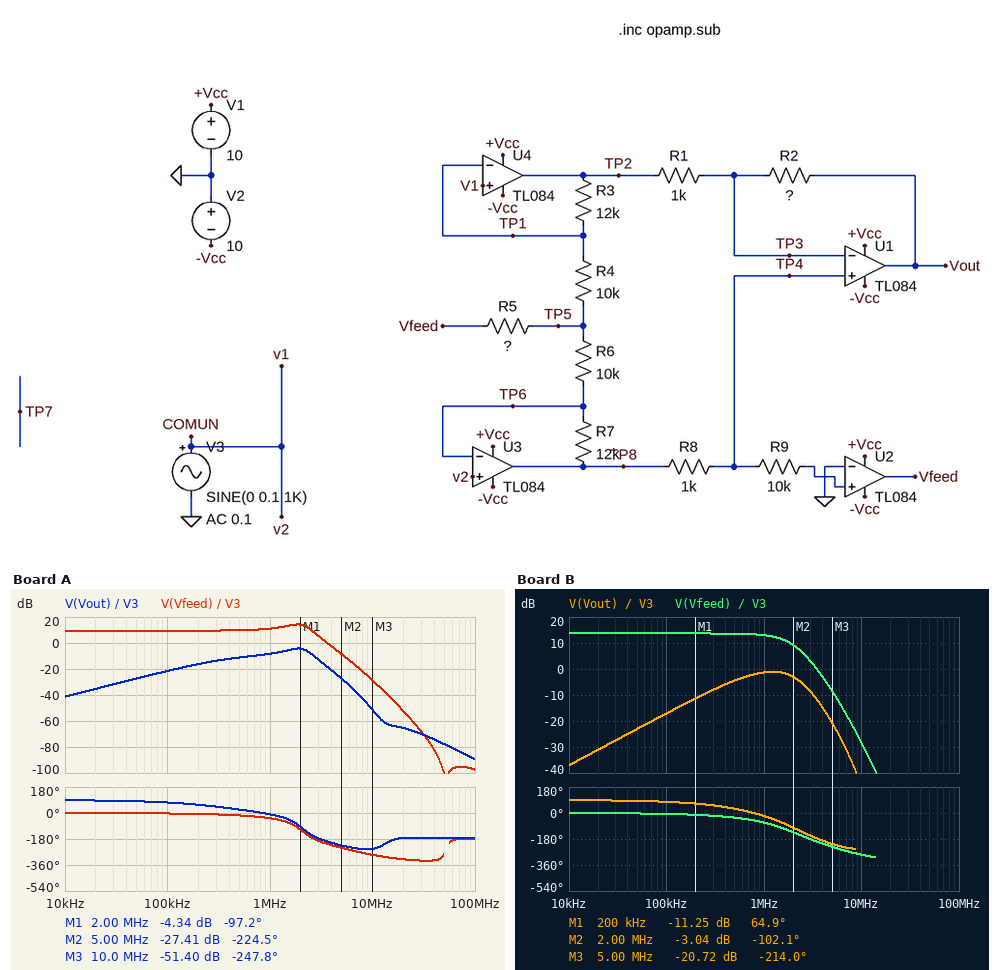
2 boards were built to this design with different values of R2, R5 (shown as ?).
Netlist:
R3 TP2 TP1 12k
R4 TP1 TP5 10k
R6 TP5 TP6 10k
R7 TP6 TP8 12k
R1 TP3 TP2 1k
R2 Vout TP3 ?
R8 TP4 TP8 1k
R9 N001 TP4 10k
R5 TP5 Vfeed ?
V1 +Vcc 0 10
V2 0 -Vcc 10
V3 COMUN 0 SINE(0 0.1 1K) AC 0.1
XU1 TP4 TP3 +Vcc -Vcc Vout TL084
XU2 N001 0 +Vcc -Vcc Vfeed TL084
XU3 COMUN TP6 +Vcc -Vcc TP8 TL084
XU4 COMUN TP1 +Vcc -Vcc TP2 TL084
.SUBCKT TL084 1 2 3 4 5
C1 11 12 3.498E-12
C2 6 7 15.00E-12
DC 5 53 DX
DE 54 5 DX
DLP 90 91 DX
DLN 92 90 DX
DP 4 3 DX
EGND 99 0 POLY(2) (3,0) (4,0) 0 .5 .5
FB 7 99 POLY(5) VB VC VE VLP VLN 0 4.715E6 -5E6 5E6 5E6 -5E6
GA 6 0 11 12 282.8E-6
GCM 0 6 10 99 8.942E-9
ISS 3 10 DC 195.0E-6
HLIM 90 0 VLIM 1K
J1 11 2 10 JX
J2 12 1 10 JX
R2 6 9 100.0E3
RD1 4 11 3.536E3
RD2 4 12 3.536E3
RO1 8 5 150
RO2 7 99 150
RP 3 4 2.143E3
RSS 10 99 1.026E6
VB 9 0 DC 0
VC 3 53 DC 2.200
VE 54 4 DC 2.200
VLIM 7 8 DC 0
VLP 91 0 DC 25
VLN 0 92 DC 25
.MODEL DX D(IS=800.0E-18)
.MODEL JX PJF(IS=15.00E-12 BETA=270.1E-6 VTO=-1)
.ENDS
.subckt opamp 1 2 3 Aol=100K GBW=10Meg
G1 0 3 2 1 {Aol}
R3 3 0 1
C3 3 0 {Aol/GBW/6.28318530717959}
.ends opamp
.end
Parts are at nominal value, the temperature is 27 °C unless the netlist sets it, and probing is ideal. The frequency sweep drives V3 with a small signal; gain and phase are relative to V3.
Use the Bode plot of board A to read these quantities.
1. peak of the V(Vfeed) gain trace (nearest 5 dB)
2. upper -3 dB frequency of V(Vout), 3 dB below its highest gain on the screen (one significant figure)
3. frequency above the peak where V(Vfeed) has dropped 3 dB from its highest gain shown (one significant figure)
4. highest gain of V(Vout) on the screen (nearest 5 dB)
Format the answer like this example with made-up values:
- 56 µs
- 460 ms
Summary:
- 15 dB
- 2 MHz
- 2 MHz
- -5 dB
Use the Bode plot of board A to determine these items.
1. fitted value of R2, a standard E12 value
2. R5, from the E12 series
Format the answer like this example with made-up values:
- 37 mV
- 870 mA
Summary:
- 8.2 kΩ
- 6.8 kΩ
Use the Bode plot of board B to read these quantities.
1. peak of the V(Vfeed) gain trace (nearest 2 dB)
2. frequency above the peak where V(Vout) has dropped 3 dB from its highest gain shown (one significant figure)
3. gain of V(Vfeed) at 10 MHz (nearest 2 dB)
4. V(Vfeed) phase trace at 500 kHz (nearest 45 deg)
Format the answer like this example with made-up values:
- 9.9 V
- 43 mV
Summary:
- 14 dB
- 2 MHz
- -28 dB
- -45 deg
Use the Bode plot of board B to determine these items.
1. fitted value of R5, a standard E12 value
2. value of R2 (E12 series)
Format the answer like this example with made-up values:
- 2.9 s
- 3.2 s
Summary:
- 18 kΩ
- 3.3 kΩ
